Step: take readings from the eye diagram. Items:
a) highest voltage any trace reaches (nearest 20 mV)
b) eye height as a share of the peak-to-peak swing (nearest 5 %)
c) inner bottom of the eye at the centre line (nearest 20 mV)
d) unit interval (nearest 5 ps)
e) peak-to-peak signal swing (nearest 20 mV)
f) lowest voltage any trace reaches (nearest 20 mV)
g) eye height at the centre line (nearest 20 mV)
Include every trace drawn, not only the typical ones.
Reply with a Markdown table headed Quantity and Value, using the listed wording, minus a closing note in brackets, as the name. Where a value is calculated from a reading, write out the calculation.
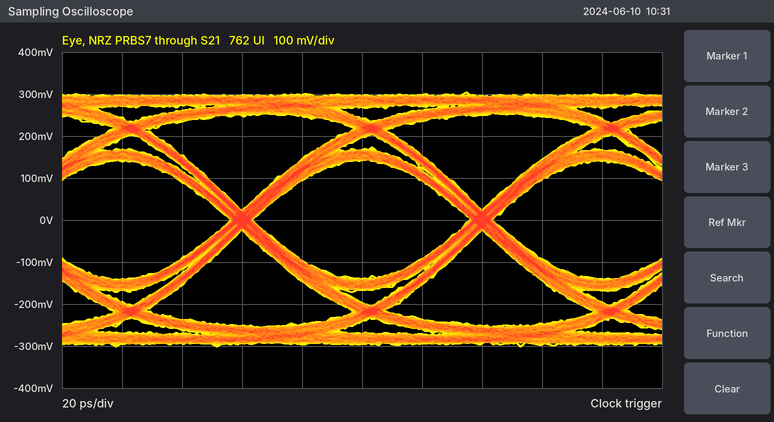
| Quantity | Value |
|---|---|
| highest voltage any trace reaches | 300 mV |
| eye height as a share of the peak-to-peak swing | 280 mV / 600 mV ≈ 46.7 %, so 45 % to the nearest 5 % |
| inner bottom of the eye at the centre line | -140 mV |
| unit interval | 80 ps |
| peak-to-peak signal swing | 600 mV |
| lowest voltage any trace reaches | -300 mV |
| eye height at the centre line | 280 mV |
